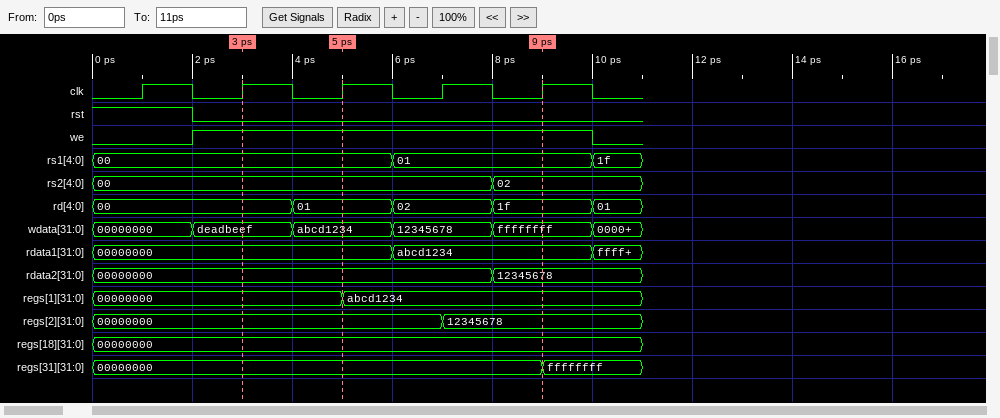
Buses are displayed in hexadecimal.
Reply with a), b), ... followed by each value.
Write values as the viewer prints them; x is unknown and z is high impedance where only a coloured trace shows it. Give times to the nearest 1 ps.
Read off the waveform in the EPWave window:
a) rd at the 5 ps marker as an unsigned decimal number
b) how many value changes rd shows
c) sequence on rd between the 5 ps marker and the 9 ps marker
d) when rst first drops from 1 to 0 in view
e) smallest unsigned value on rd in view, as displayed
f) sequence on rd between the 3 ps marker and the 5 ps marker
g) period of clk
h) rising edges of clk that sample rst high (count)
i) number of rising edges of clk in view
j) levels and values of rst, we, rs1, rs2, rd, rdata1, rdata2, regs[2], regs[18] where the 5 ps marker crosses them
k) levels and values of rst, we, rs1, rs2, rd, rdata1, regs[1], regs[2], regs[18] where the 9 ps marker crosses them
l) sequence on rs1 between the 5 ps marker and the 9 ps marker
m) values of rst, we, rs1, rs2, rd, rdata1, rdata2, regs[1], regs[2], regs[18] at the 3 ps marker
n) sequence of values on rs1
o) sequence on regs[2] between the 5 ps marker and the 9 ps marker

a) 1
b) 4
c) 01, 02, 1f
d) 2 ps
e) 00
f) 00, 01
g) 2 ps
h) 1
i) 5
j) rst=0, we=1, rs1=00, rs2=00, rd=01, rdata1=00000000, rdata2=00000000, regs[2]=00000000, regs[18]=00000000
k) rst=0, we=1, rs1=01, rs2=02, rd=1f, rdata1=abcd1234, regs[1]=abcd1234, regs[2]=12345678, regs[18]=00000000
l) 00, 01
m) rst=0, we=1, rs1=00, rs2=00, rd=00, rdata1=00000000, rdata2=00000000, regs[1]=00000000, regs[2]=00000000, regs[18]=00000000
n) 00, 01, 1f
o) 00000000, 12345678
